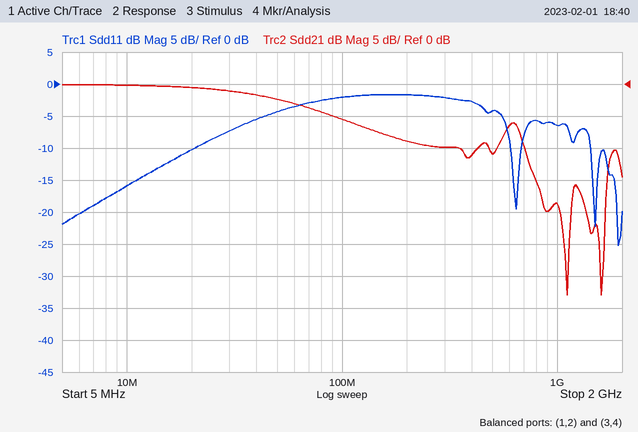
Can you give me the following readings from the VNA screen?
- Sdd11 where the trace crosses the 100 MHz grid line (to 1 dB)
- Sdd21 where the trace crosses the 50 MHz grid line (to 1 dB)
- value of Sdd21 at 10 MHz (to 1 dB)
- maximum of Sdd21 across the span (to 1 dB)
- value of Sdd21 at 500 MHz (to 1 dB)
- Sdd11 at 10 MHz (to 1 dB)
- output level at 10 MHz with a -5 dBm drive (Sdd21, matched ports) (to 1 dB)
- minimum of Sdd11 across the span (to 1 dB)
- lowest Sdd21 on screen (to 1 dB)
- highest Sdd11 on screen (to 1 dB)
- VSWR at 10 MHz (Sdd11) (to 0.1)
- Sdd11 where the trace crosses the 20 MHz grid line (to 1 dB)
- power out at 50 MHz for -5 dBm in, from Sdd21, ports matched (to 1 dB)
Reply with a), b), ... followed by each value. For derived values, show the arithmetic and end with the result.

a) -2 dB
b) -2 dB
c) 0 dB
d) 0 dB
e) -11 dB
f) -16 dB
g) -5 dBm + (0 dB) = -5 dBm
h) -25 dB
i) -33 dB
j) -2 dB
k) |Γ| = 10^(-16/20) = 0.1585; VSWR = (1 + 0.1585)/(1 − 0.1585) ≈ 1.4
l) -10 dB
m) -5 dBm + (-2 dB) = -7 dBm
